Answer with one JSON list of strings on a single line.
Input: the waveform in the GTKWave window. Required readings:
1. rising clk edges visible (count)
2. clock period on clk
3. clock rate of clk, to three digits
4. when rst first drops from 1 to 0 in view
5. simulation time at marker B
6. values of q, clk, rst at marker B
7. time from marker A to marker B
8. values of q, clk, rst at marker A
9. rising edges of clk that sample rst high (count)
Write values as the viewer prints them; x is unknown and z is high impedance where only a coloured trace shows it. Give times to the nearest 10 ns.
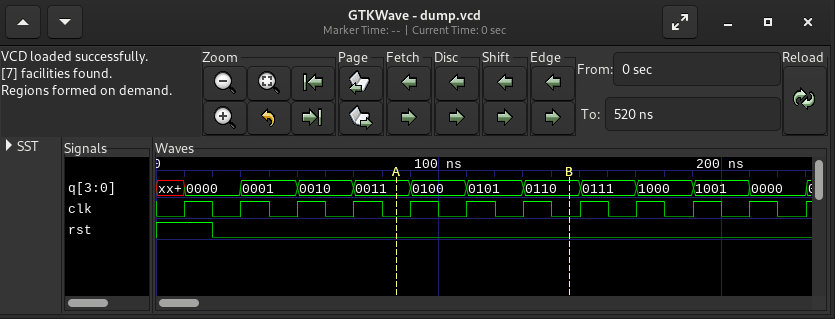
["12", "20 ns", "50.0 MHz", "20 ns", "150 ns", "q=0110, clk=0, rst=0", "60 ns", "q=0011, clk=0, rst=0", "1"]
